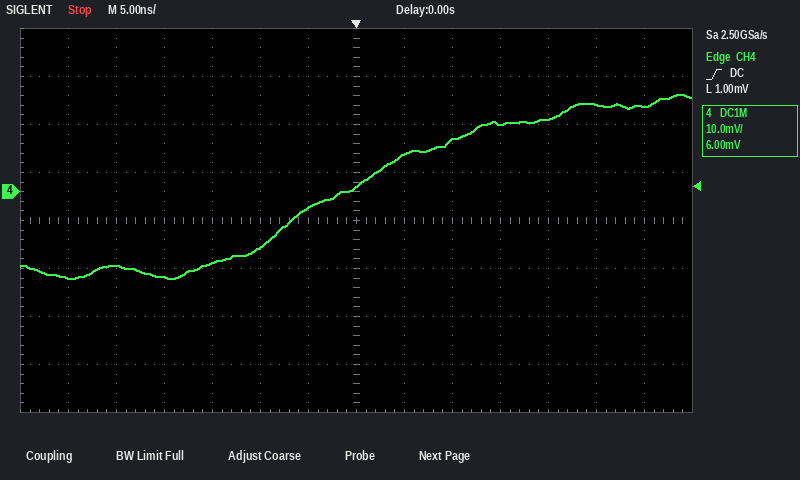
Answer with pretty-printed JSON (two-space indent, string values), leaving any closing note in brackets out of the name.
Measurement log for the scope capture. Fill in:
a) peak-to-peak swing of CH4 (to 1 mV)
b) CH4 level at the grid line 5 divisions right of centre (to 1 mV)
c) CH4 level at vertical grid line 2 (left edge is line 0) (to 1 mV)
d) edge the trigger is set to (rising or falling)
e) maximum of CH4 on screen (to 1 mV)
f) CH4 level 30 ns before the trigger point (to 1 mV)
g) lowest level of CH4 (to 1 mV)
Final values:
{
  "peak-to-peak swing of CH4": "38 mV",
  "CH4 level at the grid line 5 divisions right of centre": "18 mV",
  "CH4 level at vertical grid line 2 (left edge is line 0)": "-15 mV",
  "edge the trigger is set to": "rising",
  "maximum of CH4 on screen": "20 mV",
  "CH4 level 30 ns before the trigger point": "-18 mV",
  "lowest level of CH4": "-18 mV"
}
